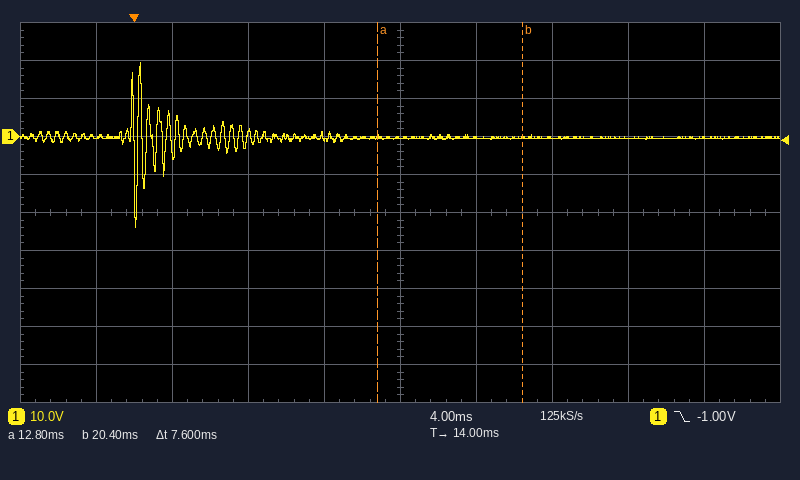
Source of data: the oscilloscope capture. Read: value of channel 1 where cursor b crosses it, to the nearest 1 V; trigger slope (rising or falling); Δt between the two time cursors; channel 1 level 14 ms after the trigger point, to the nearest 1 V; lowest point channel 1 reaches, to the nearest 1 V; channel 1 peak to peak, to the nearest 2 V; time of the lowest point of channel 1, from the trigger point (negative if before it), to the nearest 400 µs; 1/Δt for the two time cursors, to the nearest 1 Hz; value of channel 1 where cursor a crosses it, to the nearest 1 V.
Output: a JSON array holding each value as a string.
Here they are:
["0 V", "falling", "7.6 ms", "0 V", "-24 V", "44 V", "0.0 ms", "132 Hz", "0 V"]
